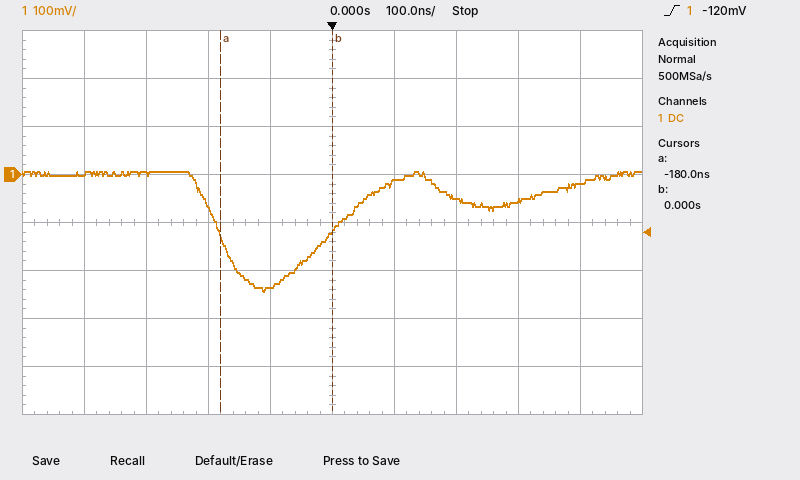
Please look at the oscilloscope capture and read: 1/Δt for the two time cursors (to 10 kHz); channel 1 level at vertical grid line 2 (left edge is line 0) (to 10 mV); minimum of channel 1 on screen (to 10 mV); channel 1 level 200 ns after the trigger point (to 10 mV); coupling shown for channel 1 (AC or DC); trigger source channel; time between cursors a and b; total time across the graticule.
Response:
5.56 MHz
0 mV
-240 mV
-50 mV
DC
channel 1
180 ns
1 µs
